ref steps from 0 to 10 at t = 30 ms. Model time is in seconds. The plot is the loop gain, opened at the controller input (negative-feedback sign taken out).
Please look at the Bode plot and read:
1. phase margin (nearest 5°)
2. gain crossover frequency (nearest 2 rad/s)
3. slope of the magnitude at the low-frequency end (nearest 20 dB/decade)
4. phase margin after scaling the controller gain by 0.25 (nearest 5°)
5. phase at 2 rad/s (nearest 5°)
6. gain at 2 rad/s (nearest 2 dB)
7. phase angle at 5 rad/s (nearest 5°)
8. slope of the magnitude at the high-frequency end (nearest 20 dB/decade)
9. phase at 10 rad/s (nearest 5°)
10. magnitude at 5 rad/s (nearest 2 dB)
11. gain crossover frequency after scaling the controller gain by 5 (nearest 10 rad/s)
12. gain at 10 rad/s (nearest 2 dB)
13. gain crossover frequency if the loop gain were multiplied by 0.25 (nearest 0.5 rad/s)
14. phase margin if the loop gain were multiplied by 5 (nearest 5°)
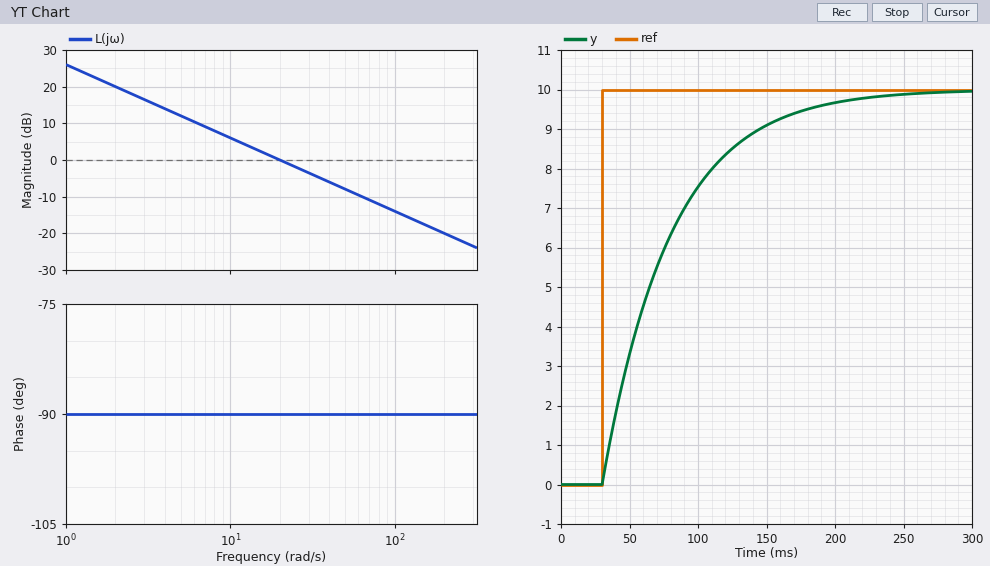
90°
20 rad/s
-20 dB/decade
90°
-90°
20 dB
-90°
-20 dB/decade
-90°
12 dB
100 rad/s
6 dB
5.0 rad/s
90°
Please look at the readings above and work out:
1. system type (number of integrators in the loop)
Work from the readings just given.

1
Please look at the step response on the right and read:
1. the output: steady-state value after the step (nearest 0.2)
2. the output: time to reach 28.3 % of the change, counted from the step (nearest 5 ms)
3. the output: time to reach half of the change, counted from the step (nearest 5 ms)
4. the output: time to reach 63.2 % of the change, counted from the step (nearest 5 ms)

10.0
15 ms
35 ms
50 ms
